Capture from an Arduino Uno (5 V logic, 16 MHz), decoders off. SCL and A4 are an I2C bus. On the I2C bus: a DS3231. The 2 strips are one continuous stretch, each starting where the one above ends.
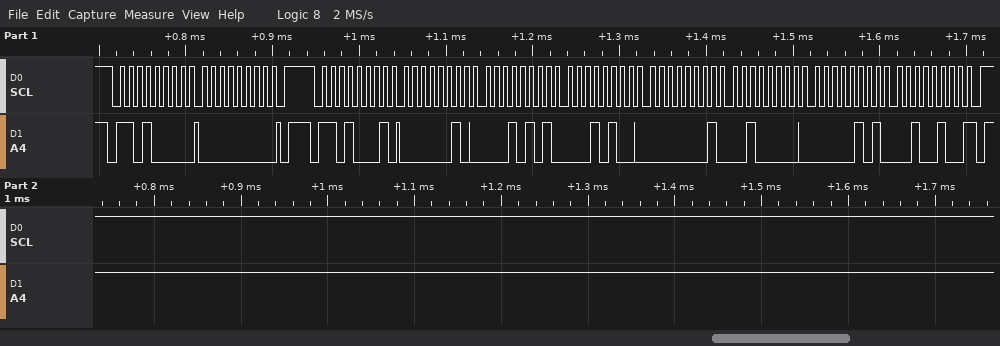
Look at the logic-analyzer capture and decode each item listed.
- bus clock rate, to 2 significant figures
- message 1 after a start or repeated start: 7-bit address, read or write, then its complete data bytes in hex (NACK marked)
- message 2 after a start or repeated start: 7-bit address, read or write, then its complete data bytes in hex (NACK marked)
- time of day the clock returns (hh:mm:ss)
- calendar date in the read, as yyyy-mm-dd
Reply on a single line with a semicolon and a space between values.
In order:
100 kHz; 0x68 write: 00; 0x68 read: 02 15 14 01 20 05 24 NACK; 14:15:02; 2024-05-20
